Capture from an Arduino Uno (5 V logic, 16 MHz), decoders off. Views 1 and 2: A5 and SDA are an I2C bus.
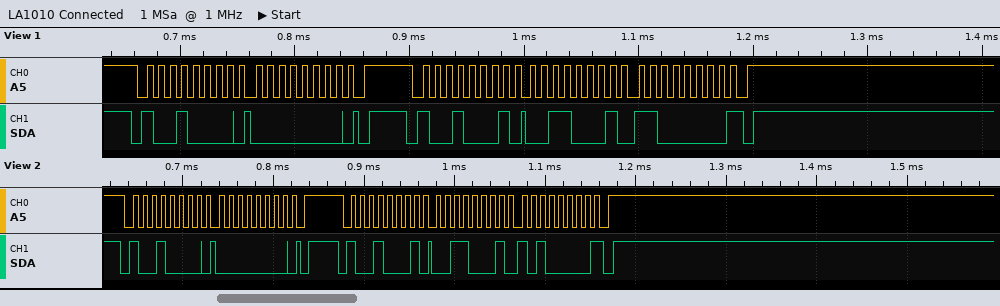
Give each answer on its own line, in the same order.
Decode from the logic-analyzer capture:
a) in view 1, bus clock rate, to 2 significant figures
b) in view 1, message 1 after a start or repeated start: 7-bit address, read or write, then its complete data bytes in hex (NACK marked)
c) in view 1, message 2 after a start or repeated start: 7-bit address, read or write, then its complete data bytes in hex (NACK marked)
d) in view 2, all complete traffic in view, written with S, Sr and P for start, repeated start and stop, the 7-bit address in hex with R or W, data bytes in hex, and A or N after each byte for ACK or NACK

100 kHz
0x48 write: 00
0x48 read: 31 C0 NACK
S 48W A 00 A P S 48R A 31 A A0 N P
